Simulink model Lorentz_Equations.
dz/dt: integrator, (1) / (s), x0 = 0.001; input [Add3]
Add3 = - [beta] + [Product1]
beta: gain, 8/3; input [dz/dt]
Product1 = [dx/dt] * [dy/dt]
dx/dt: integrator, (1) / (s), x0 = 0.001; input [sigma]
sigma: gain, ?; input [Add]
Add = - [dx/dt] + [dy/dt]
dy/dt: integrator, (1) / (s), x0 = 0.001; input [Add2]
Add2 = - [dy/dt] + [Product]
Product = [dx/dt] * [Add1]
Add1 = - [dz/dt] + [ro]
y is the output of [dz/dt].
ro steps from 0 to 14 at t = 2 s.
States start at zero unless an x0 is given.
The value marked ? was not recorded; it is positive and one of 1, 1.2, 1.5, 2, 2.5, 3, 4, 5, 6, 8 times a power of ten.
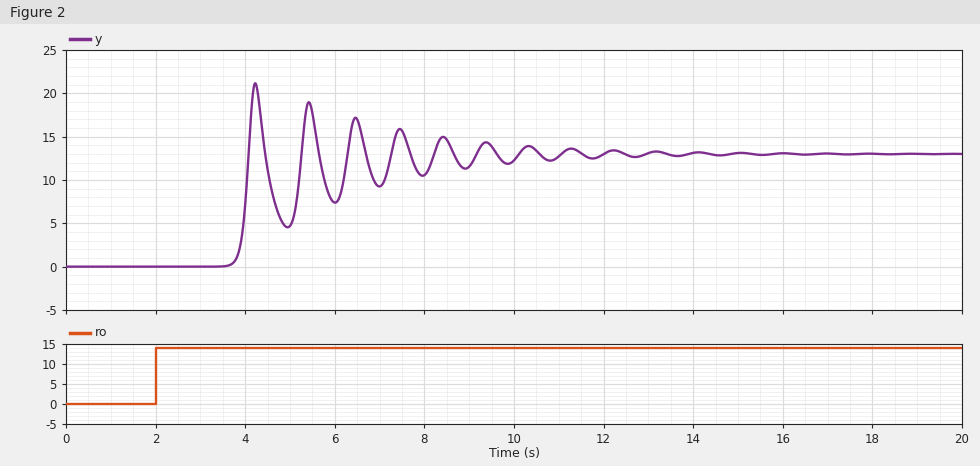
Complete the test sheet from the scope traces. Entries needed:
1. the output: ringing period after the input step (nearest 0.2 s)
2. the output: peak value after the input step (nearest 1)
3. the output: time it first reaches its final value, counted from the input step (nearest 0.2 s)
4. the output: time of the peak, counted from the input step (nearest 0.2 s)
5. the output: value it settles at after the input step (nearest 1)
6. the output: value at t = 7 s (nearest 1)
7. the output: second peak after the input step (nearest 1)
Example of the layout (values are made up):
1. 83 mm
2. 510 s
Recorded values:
1. 1.2 s
2. 21
3. 2.0 s
4. 2.2 s
5. 13
6. 9
7. 19
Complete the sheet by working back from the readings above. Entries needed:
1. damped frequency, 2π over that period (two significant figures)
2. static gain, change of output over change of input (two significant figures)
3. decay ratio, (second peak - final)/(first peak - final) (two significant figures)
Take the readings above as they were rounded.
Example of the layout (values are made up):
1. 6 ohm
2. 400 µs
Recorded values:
1. 5.2 rad/s
2. 0.93
3. 0.75
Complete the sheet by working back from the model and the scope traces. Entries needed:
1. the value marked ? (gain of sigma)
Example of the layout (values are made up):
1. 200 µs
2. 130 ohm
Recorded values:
1. 5
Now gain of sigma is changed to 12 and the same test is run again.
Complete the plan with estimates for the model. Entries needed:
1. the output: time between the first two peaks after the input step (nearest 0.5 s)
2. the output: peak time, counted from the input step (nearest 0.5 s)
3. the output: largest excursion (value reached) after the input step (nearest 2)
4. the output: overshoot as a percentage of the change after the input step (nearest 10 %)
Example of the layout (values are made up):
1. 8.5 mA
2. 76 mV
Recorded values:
1. 1.5 s
2. 1.5 s
3. 22
4. 70 %
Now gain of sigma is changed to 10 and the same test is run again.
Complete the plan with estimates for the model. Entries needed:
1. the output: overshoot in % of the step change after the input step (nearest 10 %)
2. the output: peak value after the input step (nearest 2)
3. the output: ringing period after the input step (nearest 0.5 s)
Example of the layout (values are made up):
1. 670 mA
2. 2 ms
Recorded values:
1. 70 %
2. 22
3. 1.5 s
